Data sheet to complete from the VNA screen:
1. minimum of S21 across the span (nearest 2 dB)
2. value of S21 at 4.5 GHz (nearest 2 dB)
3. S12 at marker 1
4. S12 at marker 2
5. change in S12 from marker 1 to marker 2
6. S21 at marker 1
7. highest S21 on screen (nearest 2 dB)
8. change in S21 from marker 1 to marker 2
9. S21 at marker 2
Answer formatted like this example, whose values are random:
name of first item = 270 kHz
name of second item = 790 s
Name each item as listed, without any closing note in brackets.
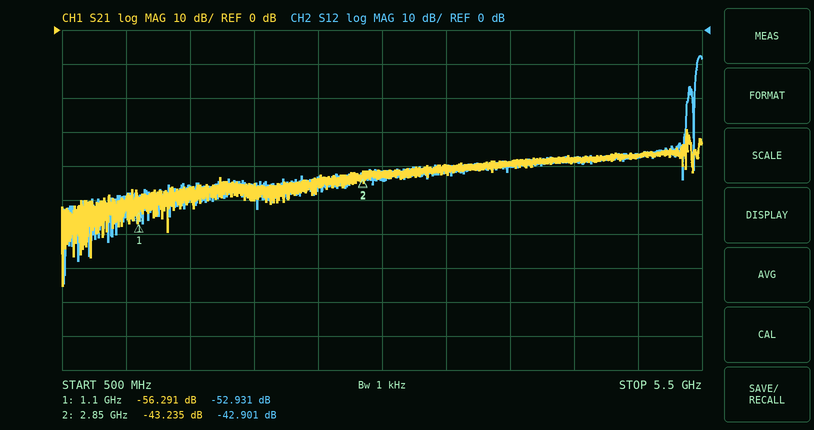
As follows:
minimum of S21 across the span = -76 dB
value of S21 at 4.5 GHz = -38 dB
S12 at marker 1 = -52.931 dB
S12 at marker 2 = -42.901 dB
change in S12 from marker 1 to marker 2 = 10.030 dB
S21 at marker 1 = -56.291 dB
highest S21 on screen = -30 dB
change in S21 from marker 1 to marker 2 = 13.056 dB
S21 at marker 2 = -43.235 dB
